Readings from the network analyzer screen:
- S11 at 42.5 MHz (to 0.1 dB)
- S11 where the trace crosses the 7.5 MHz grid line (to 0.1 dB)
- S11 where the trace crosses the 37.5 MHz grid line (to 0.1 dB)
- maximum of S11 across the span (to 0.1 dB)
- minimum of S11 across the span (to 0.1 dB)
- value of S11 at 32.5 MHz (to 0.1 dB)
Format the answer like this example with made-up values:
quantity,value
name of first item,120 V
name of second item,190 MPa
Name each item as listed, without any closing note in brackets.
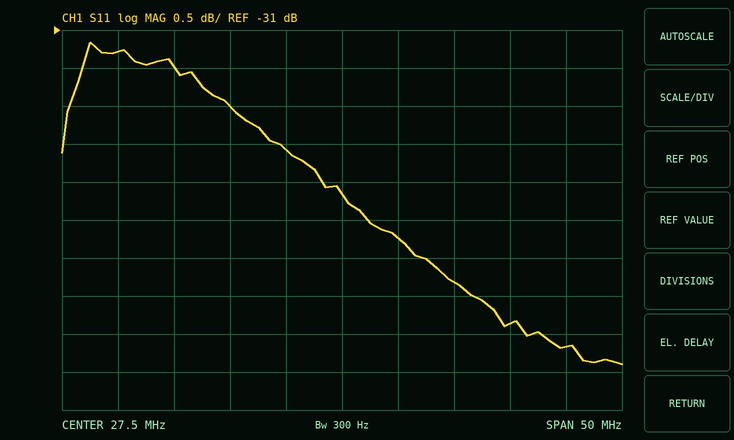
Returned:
quantity,value
S11 at 42.5 MHz,-34.9 dB
S11 where the trace crosses the 7.5 MHz grid line,-31.3 dB
S11 where the trace crosses the 37.5 MHz grid line,-34.3 dB
maximum of S11 across the span,-31.2 dB
minimum of S11 across the span,-35.4 dB
value of S11 at 32.5 MHz,-33.7 dB
